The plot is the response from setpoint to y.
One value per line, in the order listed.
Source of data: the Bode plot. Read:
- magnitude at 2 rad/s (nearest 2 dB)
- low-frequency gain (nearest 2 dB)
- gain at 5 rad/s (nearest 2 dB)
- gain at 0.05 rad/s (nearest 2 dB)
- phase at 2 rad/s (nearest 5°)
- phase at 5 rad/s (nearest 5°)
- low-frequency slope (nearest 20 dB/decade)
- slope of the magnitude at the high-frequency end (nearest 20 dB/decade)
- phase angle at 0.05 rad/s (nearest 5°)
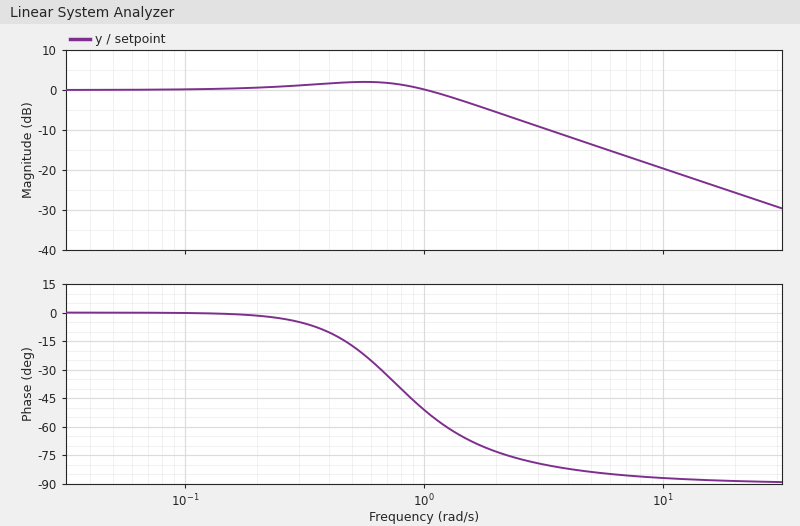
-6 dB
0 dB
-14 dB
0 dB
-75°
-85°
0 dB/decade
-20 dB/decade
0°
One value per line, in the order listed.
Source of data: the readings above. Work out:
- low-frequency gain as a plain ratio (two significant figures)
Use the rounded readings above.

1.0
